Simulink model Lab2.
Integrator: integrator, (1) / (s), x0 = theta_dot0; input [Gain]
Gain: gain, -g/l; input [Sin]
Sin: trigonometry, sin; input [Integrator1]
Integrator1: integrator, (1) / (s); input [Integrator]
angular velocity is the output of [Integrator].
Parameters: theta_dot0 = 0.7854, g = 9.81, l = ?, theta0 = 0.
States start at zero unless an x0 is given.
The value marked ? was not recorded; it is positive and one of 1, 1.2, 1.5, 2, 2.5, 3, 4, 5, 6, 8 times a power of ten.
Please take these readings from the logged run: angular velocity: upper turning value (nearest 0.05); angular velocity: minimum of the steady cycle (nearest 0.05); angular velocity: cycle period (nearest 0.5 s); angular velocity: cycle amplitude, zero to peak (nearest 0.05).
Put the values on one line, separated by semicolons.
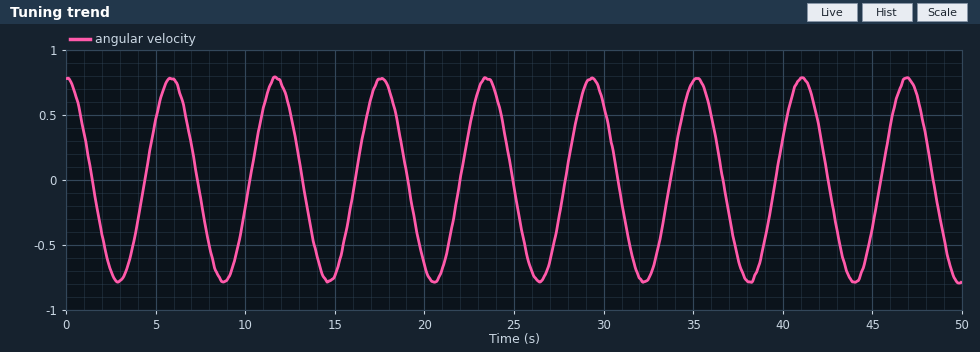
0.80; -0.80; 6.0 s; 0.80
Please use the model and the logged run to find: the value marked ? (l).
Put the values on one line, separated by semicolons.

8
